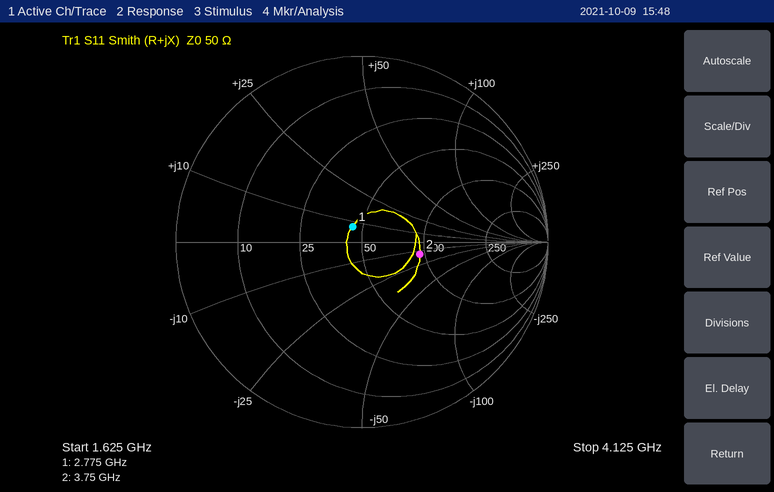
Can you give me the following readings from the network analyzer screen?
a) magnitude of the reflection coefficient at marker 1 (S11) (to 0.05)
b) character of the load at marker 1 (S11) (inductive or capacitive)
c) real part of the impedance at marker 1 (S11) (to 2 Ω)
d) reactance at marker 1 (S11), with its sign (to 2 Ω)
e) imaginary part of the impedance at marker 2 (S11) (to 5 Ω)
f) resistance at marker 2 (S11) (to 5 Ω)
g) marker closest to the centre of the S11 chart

0.10
inductive
44 Ω
+8 Ω
-15 Ω
95 Ω
marker 1
